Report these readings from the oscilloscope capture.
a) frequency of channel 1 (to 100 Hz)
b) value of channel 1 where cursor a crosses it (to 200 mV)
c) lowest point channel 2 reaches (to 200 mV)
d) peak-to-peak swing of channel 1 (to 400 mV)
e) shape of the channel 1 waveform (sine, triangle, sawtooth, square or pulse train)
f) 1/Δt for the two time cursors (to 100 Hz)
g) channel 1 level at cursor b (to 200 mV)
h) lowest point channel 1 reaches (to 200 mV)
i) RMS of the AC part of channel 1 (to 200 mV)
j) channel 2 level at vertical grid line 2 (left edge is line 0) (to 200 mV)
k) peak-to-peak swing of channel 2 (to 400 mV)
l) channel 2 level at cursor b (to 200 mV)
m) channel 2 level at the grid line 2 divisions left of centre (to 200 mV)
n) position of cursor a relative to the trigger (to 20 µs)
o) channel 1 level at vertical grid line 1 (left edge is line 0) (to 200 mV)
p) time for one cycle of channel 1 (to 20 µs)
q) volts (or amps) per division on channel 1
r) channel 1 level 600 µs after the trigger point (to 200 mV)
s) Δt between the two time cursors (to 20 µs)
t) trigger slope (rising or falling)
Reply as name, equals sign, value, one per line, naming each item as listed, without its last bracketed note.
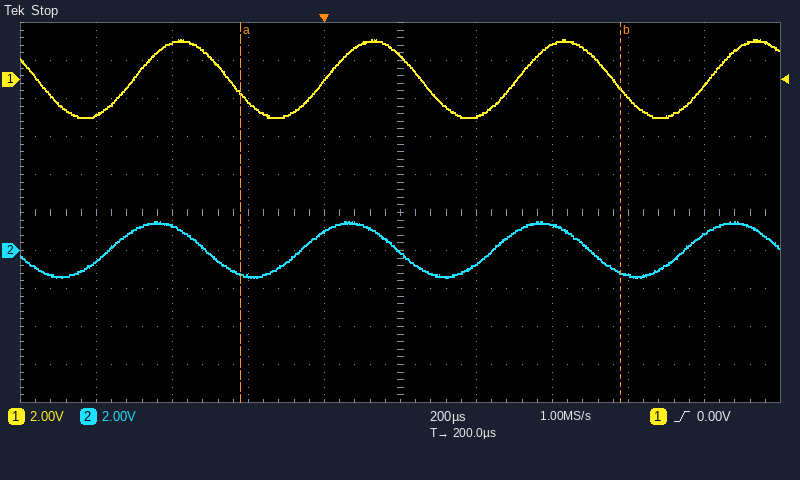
frequency of channel 1 = 2.0 kHz
value of channel 1 where cursor a crosses it = -800 mV
lowest point channel 2 reaches = -1.4 V
peak-to-peak swing of channel 1 = 4.0 V
shape of the channel 1 waveform = sine
1/Δt for the two time cursors = 1.0 kHz
channel 1 level at cursor b = -400 mV
lowest point channel 1 reaches = -2.0 V
RMS of the AC part of channel 1 = 1.4 V
channel 2 level at vertical grid line 2 (left edge is line 0) = 1.4 V
peak-to-peak swing of channel 2 = 2.8 V
channel 2 level at cursor b = -1.2 V
channel 2 level at the grid line 2 divisions left of centre = -1.4 V
position of cursor a relative to the trigger = -220 µs
channel 1 level at vertical grid line 1 (left edge is line 0) = -1.8 V
time for one cycle of channel 1 = 500 µs
volts (or amps) per division on channel 1 = 2 V
channel 1 level 600 µs after the trigger point = 1.8 V
Δt between the two time cursors = 1.00 ms
trigger slope = rising
